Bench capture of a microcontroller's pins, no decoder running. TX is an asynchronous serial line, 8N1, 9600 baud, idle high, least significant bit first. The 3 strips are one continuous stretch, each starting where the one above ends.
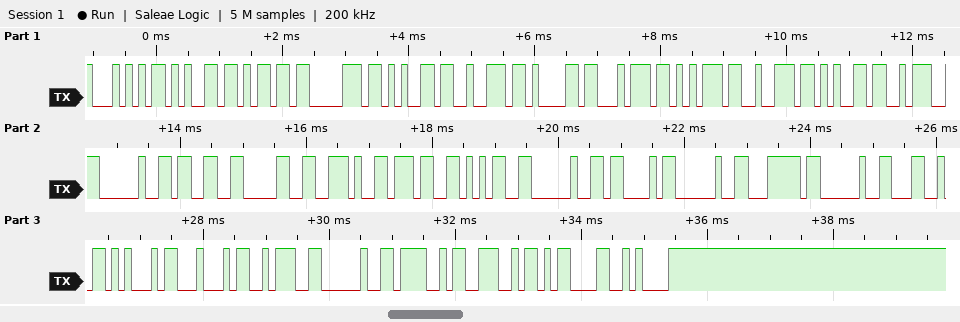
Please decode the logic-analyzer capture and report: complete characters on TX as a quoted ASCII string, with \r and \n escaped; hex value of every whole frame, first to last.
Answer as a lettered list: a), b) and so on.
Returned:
a) "Temperature: 30.75 C | LED: ON\r\n"
b) 54 65 6D 70 65 72 61 74 75 72 65 3A 20 33 30 2E 37 35 20 43 20 7C 20 4C 45 44 3A 20 4F 4E 0D 0A
